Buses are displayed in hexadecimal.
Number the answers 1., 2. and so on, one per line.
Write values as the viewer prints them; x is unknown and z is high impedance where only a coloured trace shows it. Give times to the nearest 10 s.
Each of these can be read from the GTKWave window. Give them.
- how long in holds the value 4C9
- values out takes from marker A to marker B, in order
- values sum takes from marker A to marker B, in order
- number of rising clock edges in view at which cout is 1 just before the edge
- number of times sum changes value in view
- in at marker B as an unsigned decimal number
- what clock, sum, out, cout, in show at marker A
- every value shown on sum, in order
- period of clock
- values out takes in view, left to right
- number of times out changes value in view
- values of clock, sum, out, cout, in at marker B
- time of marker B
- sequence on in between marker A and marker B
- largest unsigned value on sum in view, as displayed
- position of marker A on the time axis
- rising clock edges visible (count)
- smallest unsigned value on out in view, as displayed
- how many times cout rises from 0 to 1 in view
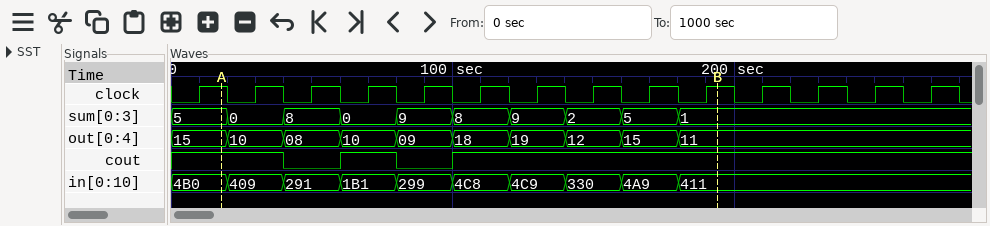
1. 20 s
2. 15, 10, 08, 10, 09, 18, 19, 12, 15, 11
3. 5, 0, 8, 0, 9, 8, 9, 2, 5, 1
4. 12
5. 9
6. 1041
7. clock=1, sum=5, out=15, cout=1, in=4B0
8. 5, 0, 8, 0, 9, 8, 9, 2, 5, 1
9. 20 s
10. 15, 10, 08, 10, 09, 18, 19, 12, 15, 11
11. 9
12. clock=1, sum=1, out=11, cout=1, in=411
13. 190 s
14. 4B0, 409, 291, 1B1, 299, 4C8, 4C9, 330, 4A9, 411
15. 9
16. 20 s
17. 14
18. 08
19. 2
